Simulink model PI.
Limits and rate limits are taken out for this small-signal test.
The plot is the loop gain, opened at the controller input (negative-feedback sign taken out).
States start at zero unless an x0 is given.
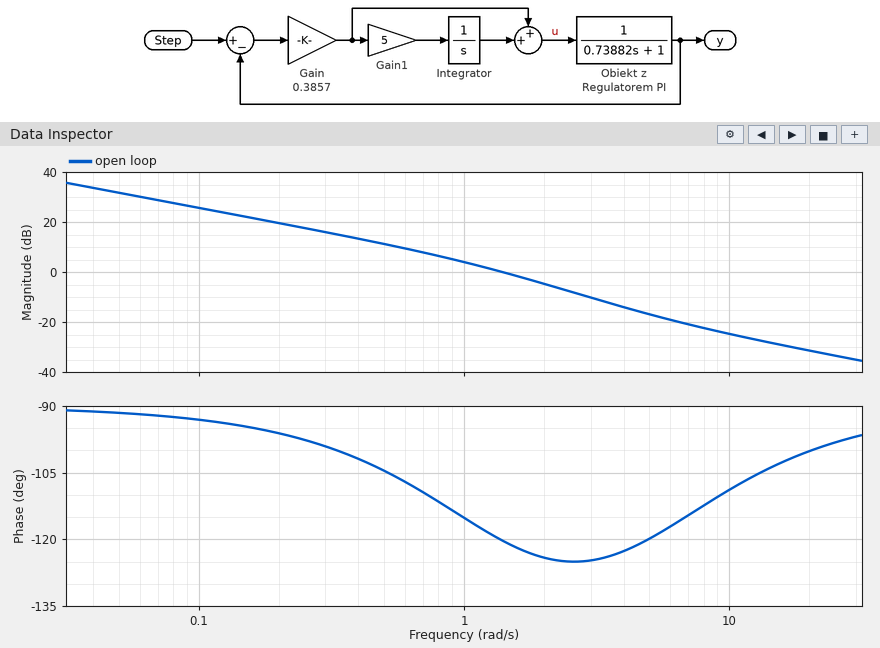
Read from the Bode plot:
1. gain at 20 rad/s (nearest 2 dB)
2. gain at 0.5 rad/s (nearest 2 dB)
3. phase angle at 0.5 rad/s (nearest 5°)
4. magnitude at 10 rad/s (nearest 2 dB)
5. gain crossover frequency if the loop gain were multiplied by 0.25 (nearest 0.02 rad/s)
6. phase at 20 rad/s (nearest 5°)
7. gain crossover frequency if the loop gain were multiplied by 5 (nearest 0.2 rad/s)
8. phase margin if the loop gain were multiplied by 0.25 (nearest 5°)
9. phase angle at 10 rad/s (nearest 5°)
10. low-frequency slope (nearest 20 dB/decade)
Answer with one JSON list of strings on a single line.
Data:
["-32 dB", "12 dB", "-105°", "-24 dB", "0.46 rad/s", "-100°", "4.0 rad/s", "75°", "-110°", "-20 dB/decade"]
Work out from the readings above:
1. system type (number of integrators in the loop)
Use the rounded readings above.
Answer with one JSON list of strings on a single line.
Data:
["1"]
